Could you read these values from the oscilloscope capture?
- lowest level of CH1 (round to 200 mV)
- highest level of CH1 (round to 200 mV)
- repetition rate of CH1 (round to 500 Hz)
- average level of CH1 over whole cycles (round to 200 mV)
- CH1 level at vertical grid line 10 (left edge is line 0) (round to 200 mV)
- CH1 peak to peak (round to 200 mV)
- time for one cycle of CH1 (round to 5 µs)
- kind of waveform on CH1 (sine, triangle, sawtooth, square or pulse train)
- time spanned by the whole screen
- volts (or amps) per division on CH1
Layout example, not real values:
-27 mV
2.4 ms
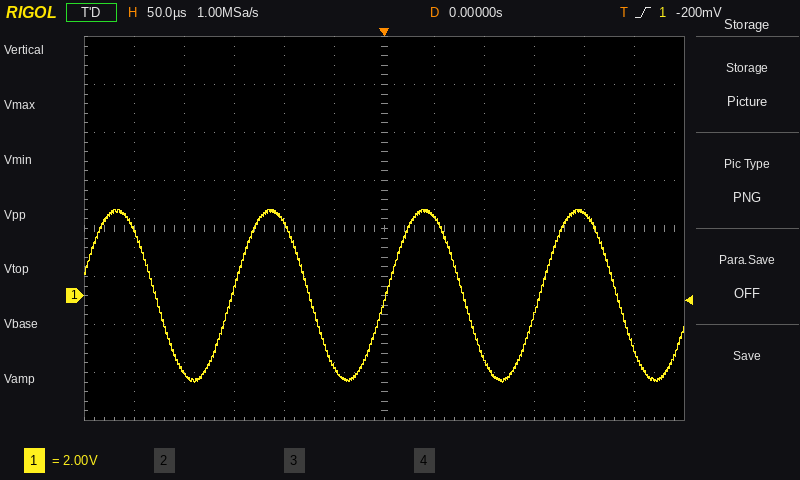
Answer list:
-3.6 V
3.6 V
6.5 kHz
0.0 V
3.4 V
7.2 V
155 µs
sine
600 µs
2 V
